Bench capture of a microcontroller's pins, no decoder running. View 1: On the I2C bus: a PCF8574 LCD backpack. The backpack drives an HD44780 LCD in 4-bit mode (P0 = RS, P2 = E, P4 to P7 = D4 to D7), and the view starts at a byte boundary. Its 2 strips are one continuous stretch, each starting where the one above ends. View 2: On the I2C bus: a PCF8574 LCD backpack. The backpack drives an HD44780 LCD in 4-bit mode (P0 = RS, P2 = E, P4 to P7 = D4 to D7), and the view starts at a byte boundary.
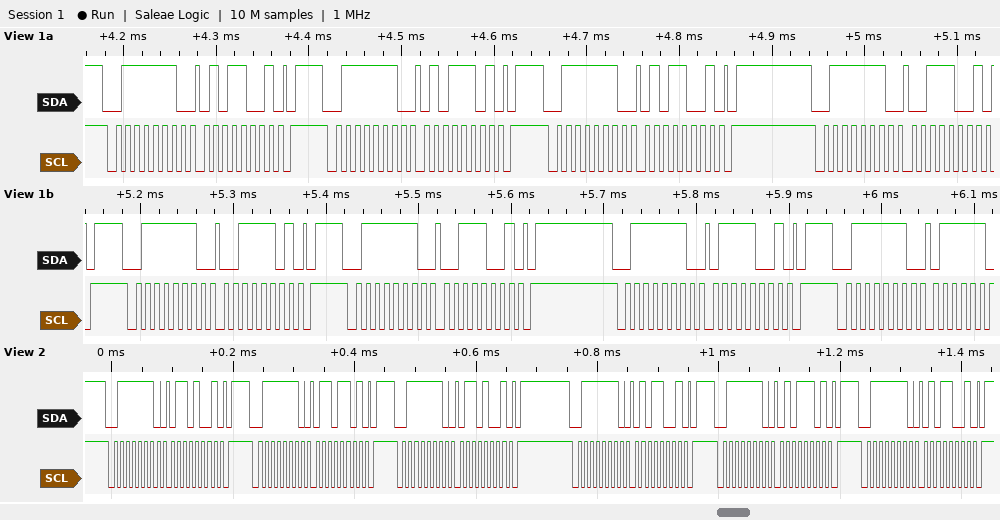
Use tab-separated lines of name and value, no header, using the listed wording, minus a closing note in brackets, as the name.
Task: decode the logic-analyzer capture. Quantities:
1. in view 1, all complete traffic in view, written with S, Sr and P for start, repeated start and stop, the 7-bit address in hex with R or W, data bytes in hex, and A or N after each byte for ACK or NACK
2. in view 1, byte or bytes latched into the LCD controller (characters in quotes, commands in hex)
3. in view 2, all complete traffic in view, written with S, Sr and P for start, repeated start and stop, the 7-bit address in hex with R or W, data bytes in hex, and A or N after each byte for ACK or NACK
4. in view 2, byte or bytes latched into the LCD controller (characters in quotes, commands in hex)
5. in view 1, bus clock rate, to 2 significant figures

in view 1, all complete traffic in view, written with S, Sr and P for start, repeated start and stop, the 7-bit address in hex with R or W, data bytes in hex, and A or N after each byte for ACK or NACK	S 3FW A 59 A P S 3FW A 5D A P S 3FW A 59 A P S 3FW A 39 A P S 3FW A 3D A P S 3FW A 39 A P S 3FW A 79 A P S 3FW A
in view 1, byte or bytes latched into the LCD controller	'S'
in view 2, all complete traffic in view, written with S, Sr and P for start, repeated start and stop, the 7-bit address in hex with R or W, data bytes in hex, and A or N after each byte for ACK or NACK	S 3FW A 69 A P S 3FW A 6D A P S 3FW A 69 A P S 3FW A 59 A P S 3FW A 5D A P S 3FW A 59 A P
in view 2, byte or bytes latched into the LCD controller	'e'
in view 1, bus clock rate, to 2 significant figures	100 kHz
